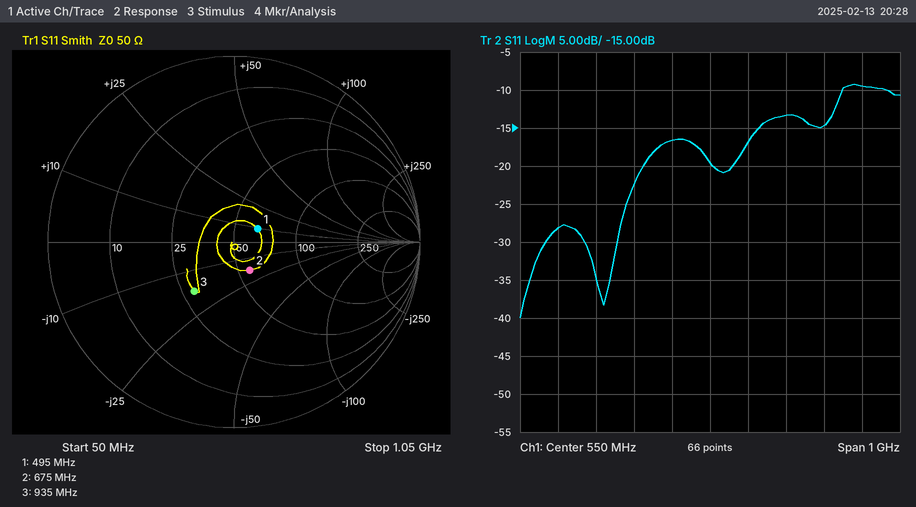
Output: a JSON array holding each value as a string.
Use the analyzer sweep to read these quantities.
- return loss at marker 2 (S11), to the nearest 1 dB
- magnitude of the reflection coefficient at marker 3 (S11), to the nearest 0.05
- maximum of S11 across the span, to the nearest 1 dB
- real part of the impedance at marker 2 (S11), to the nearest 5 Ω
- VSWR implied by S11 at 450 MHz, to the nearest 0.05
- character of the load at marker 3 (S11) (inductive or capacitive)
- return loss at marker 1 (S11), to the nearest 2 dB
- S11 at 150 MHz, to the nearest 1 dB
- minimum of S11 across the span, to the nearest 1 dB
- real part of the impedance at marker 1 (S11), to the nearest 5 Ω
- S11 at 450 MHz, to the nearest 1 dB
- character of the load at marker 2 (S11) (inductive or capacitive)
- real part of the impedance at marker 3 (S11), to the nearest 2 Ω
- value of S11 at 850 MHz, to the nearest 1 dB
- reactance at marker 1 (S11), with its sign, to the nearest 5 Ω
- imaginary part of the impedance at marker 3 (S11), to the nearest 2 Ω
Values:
["15 dB", "0.35", "-9 dB", "55 Ω", "1.35", "capacitive", "16 dB", "-28 dB", "-40 dB", "65 Ω", "-17 dB", "capacitive", "28 Ω", "-15 dB", "+10 Ω", "-18 Ω"]
